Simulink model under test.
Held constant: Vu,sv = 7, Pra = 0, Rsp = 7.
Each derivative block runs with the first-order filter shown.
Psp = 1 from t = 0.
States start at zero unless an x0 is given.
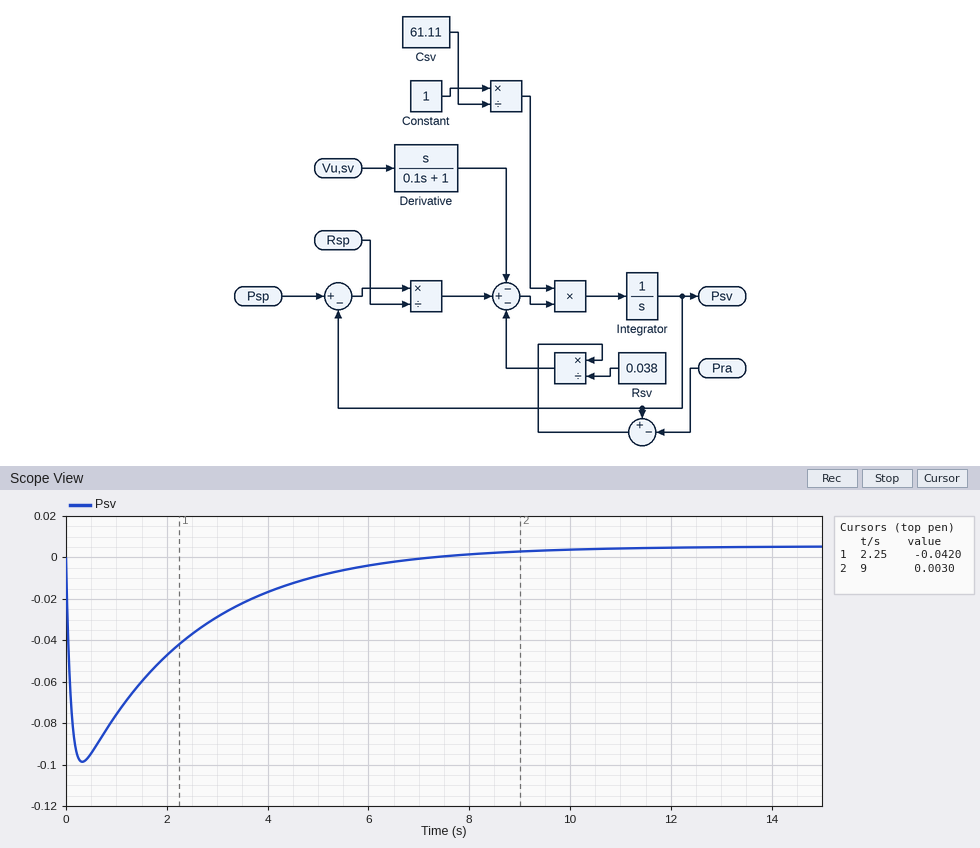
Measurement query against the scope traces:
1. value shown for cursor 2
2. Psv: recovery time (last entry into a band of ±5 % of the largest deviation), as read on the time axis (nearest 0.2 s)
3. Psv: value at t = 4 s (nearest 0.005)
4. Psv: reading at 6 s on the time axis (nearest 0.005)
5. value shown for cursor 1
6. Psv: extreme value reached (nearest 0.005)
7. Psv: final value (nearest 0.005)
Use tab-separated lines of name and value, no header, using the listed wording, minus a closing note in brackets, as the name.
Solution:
value shown for cursor 2	0.0030
Psv: recovery time (last entry into a band of ±5 % of the largest deviation), as read on the time axis	7.4 s
Psv: value at t = 4 s	-0.015
Psv: reading at 6 s on the time axis	-0.005
value shown for cursor 1	-0.0420
Psv: extreme value reached	-0.100
Psv: final value	0.005
